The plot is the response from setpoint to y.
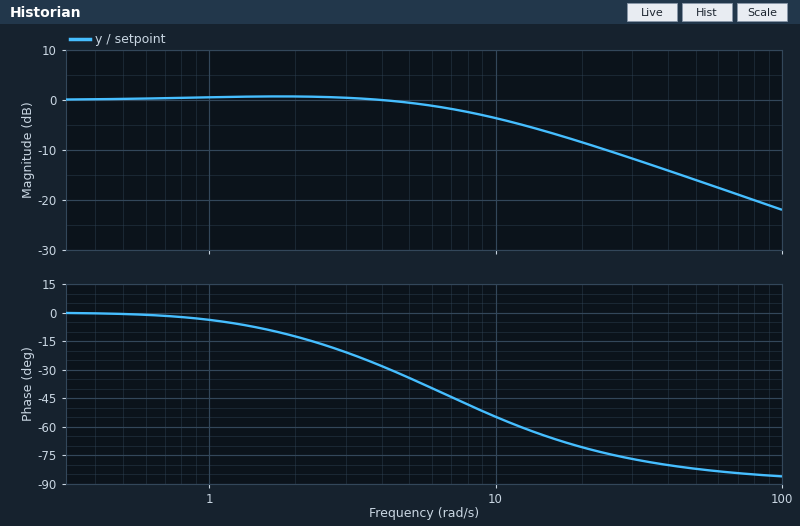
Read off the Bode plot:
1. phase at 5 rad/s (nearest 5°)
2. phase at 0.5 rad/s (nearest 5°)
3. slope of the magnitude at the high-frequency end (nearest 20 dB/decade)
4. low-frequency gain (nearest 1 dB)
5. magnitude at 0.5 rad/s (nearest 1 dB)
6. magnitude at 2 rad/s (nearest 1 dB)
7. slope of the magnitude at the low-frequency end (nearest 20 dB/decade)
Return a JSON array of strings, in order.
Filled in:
["-35°", "0°", "-20 dB/decade", "0 dB", "0 dB", "1 dB", "0 dB/decade"]
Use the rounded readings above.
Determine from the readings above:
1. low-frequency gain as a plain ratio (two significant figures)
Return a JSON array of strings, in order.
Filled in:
["1.0"]
